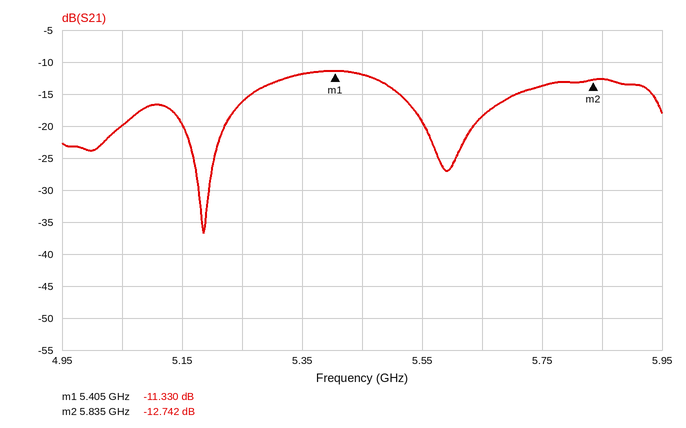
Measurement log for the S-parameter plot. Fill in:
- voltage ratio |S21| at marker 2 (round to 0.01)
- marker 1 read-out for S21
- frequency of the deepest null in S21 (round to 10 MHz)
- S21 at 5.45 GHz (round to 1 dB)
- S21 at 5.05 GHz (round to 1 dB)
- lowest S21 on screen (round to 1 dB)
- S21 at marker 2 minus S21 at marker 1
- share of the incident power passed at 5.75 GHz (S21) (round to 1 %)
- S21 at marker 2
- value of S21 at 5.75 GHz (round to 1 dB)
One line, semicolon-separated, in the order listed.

0.23; -11.330 dB; 5.19 GHz; -12 dB; -20 dB; -37 dB; -1.412 dB; 4 %; -12.742 dB; -14 dB
